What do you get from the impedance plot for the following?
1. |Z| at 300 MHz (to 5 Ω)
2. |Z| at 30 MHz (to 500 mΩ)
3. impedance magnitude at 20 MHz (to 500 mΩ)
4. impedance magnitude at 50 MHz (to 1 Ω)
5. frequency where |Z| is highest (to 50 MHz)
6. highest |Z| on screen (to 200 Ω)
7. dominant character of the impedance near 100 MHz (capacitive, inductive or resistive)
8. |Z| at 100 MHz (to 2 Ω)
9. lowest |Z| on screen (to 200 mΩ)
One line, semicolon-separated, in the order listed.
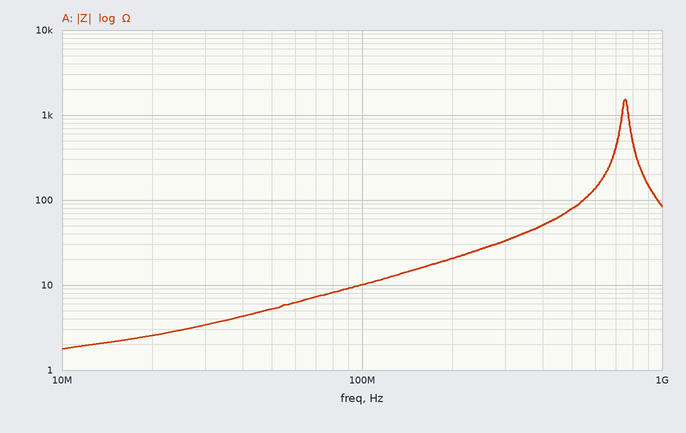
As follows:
35 Ω; 3.5 Ω; 2.5 Ω; 5 Ω; 750 MHz; 1.6 kΩ; inductive; 10 Ω; 1.8 Ω
